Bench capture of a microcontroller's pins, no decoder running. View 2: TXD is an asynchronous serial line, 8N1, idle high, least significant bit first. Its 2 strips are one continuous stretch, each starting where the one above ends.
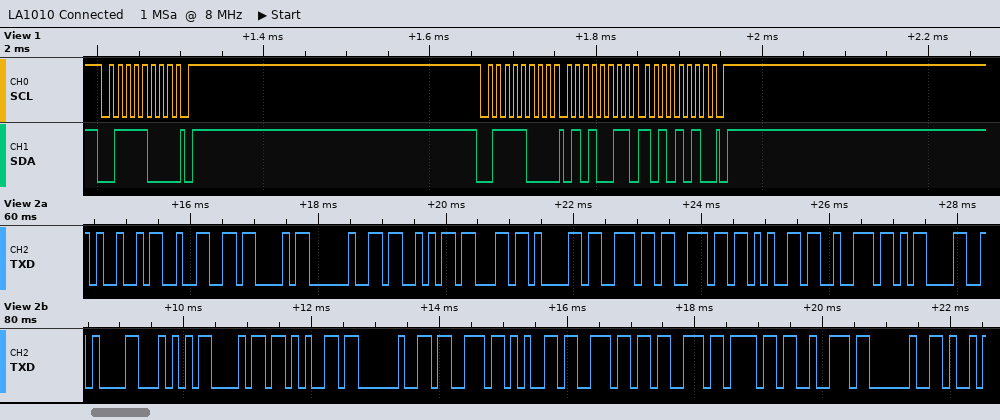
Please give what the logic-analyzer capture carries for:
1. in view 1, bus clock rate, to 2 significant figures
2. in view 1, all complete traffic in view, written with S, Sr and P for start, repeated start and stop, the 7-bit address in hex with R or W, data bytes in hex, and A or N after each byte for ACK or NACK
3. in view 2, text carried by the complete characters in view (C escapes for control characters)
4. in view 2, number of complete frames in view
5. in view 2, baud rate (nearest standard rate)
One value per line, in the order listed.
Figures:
100 kHz
S 3CW A P S 3CW A 53 A AA A P
"I2C Scanner\r\nThe sensor "
24
9600 baud
